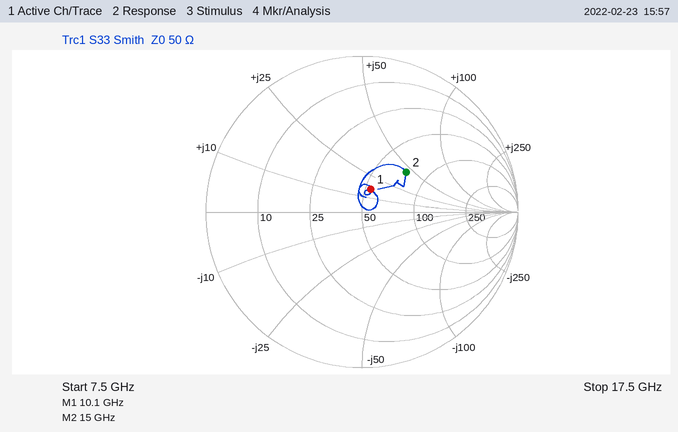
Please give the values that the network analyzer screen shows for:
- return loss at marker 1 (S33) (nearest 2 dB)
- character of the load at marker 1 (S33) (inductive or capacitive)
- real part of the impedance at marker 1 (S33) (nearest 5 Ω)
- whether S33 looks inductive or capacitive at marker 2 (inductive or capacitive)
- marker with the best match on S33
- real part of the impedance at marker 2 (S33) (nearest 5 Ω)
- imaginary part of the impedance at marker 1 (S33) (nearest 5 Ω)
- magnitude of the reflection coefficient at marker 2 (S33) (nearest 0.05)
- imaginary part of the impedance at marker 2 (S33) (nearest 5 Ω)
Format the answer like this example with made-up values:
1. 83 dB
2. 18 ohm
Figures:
1. 16 dB
2. inductive
3. 55 Ω
4. inductive
5. marker 1
6. 75 Ω
7. +15 Ω
8. 0.40
9. +45 Ω
